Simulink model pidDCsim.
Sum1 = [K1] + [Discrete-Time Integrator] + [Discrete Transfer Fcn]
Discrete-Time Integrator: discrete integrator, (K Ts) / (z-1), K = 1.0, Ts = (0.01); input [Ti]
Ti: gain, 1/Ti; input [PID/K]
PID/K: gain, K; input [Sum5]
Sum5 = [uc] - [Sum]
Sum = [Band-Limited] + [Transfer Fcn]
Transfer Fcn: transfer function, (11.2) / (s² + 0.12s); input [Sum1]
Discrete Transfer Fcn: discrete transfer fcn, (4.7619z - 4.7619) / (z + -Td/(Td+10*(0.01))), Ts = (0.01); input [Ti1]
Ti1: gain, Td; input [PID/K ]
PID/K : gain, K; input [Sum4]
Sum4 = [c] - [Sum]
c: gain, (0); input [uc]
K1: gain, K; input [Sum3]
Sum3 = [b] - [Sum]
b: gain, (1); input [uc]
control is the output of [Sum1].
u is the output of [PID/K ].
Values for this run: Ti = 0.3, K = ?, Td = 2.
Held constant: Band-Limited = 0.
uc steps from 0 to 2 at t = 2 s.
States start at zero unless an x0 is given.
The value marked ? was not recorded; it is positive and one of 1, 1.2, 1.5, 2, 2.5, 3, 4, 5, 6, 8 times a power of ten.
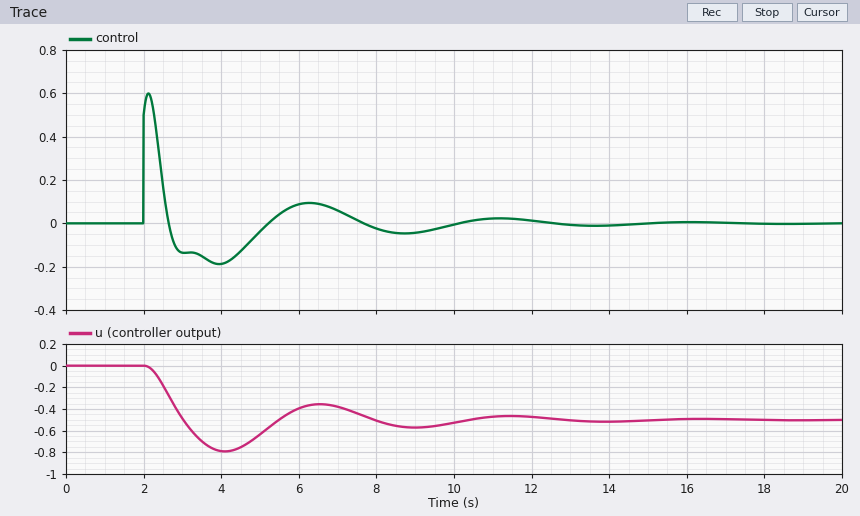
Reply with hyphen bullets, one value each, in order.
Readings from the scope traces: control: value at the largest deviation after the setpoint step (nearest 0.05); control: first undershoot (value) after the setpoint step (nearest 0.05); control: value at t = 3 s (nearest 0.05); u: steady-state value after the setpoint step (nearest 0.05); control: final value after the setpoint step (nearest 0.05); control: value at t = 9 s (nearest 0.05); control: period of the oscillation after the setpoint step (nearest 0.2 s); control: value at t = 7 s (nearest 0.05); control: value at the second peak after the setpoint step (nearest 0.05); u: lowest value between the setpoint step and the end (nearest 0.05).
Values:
- 0.60
- -0.20
- -0.15
- -0.50
- 0.00
- -0.05
- 4.2 s
- 0.05
- 0.10
- -0.80
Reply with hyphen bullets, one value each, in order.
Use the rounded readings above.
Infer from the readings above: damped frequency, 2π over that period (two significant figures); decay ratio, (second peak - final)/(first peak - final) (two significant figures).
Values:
- 1.5 rad/s
- 0.17
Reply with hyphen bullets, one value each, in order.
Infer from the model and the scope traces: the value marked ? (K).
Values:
- 0.25
